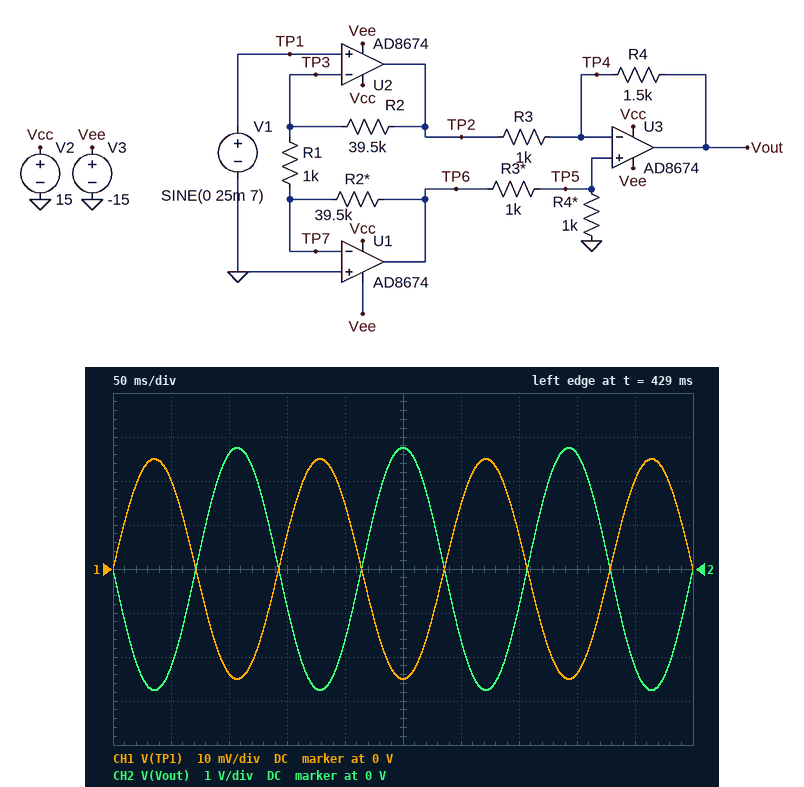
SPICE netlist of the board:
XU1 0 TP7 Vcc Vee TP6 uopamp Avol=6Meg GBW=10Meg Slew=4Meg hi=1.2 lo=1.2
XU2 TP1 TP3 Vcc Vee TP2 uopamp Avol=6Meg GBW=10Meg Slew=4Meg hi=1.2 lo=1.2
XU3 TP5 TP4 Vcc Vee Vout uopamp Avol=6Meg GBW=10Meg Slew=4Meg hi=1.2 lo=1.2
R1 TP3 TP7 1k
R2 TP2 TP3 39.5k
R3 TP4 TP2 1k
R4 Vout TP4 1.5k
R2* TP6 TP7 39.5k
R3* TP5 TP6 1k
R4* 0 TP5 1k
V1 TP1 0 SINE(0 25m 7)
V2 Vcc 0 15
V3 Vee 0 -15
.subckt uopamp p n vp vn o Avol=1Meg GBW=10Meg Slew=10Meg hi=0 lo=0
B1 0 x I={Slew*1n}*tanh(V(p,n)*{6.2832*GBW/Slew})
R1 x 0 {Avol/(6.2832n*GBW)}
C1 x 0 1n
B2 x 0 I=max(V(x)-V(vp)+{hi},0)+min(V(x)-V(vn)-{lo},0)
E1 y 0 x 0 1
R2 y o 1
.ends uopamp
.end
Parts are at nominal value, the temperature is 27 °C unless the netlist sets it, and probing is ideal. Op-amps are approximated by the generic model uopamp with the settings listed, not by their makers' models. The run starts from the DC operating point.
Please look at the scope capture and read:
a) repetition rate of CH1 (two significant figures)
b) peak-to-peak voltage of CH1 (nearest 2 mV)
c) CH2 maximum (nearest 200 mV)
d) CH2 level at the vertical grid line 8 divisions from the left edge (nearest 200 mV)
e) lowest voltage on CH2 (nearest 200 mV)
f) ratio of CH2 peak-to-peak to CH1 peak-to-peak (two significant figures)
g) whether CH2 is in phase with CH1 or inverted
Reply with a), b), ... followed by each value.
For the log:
a) 7.0 Hz
b) 50 mV
c) 2.8 V
d) 2.6 V
e) -2.8 V
f) 110
g) inverted
